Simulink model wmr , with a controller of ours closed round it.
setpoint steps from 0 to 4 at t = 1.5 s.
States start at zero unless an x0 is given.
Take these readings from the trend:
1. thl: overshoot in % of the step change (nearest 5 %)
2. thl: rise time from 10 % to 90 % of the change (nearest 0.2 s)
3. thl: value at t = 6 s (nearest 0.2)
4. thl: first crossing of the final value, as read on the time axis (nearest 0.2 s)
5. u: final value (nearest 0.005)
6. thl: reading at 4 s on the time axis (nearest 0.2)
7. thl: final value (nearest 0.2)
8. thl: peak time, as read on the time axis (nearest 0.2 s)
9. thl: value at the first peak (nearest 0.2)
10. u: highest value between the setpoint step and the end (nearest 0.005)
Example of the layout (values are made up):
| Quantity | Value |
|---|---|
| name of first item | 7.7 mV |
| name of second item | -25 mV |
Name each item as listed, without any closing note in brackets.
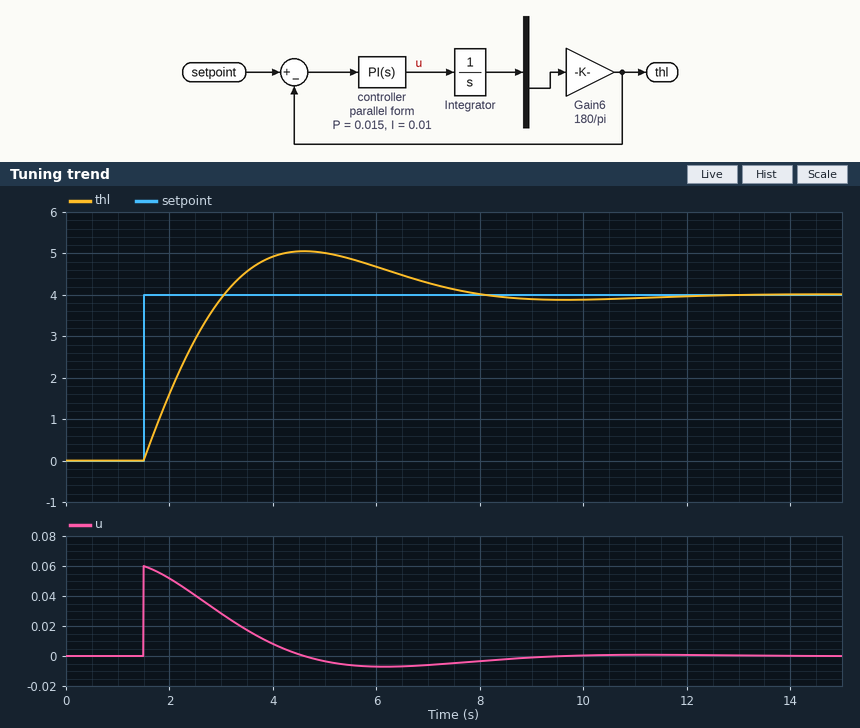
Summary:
| Quantity | Value |
|---|---|
| thl: overshoot in % of the step change | 25 % |
| thl: rise time from 10 % to 90 % of the change | 1.2 s |
| thl: value at t = 6 s | 4.6 |
| thl: first crossing of the final value, as read on the time axis | 3.0 s |
| u: final value | 0.000 |
| thl: reading at 4 s on the time axis | 5.0 |
| thl: final value | 4.0 |
| thl: peak time, as read on the time axis | 4.6 s |
| thl: value at the first peak | 5.0 |
| u: highest value between the setpoint step and the end | 0.060 |
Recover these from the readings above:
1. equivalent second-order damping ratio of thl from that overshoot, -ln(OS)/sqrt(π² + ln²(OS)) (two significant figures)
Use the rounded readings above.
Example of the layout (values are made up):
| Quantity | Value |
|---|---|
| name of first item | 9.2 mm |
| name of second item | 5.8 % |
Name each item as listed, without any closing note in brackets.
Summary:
| Quantity | Value |
|---|---|
| equivalent second-order damping ratio of thl from that overshoot, -ln(OS)/sqrt(π² + ln²(OS)) | 0.40 |
